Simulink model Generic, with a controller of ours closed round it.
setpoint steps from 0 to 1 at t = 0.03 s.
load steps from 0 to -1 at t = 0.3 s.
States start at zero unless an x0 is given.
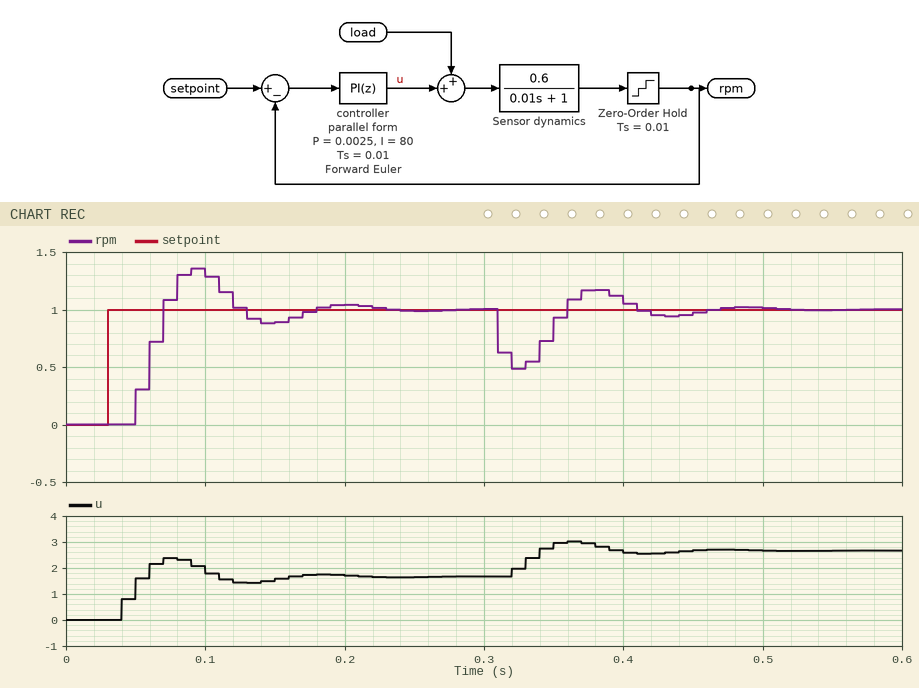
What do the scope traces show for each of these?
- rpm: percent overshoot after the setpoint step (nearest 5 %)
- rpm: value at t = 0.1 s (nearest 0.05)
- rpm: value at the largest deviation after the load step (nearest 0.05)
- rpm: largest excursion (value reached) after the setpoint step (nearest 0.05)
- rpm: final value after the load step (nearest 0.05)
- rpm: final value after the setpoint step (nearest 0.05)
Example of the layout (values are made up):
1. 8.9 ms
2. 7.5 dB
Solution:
1. 35 %
2. 1.30
3. 0.50
4. 1.35
5. 1.00
6. 1.00
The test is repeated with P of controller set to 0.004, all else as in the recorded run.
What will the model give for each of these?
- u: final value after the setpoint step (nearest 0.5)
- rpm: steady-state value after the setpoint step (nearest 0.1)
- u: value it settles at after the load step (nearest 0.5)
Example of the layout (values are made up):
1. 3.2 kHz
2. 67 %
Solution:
1. 1.5
2. 1.0
3. 2.5
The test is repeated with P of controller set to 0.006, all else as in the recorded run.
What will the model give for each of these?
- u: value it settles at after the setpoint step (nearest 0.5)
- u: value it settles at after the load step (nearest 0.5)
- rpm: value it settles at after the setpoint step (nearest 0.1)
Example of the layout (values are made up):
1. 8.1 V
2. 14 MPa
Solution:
1. 1.5
2. 2.5
3. 1.0
